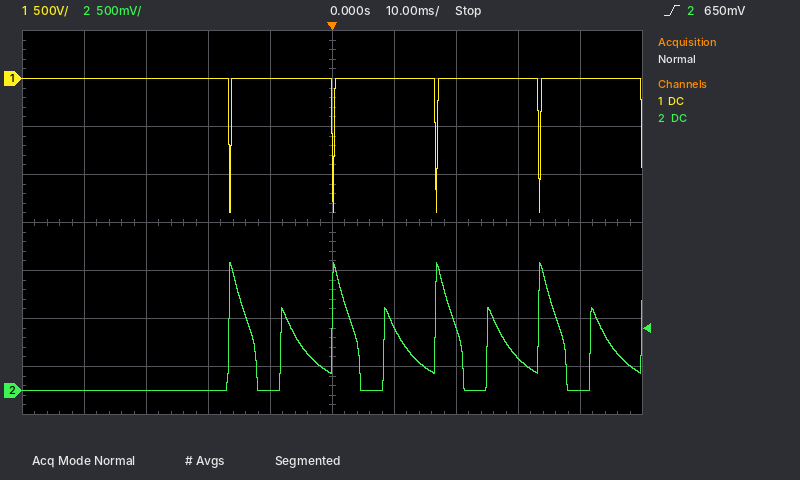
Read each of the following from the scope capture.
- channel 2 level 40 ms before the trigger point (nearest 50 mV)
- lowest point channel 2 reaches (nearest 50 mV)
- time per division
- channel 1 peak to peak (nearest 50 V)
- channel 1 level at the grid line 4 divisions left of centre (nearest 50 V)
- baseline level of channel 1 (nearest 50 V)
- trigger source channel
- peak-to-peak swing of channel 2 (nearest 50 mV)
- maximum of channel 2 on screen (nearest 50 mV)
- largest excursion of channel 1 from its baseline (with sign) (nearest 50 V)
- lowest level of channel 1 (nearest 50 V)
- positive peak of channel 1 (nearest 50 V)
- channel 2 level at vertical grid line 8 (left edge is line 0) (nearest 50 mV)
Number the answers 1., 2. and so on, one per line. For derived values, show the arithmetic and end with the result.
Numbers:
1. 0 mV
2. 0 mV
3. 10 ms
4. 0 V − (-1.40 kV) = 1.40 kV
5. 0 V
6. 0 V
7. channel 2
8. 1.35 V − (0 mV) = 1.35 V
9. 1.35 V
10. -1.40 kV − (0 V) = -1.40 kV
11. -1.40 kV
12. 0 V
13. 350 mV
